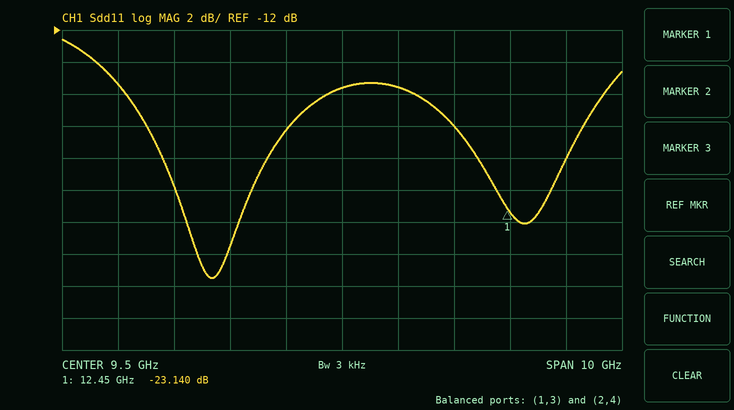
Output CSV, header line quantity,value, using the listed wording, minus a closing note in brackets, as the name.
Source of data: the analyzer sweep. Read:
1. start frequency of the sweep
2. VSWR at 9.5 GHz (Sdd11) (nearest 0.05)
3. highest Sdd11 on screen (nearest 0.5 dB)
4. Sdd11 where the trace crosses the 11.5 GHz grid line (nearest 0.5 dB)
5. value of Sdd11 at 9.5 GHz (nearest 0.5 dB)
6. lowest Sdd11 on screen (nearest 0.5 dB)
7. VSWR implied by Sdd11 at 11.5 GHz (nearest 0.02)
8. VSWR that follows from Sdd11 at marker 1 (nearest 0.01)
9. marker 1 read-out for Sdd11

quantity,value
start frequency of the sweep,4.5 GHz
VSWR at 9.5 GHz (Sdd11),1.40
highest Sdd11 on screen,-12.5 dB
Sdd11 where the trace crosses the 11.5 GHz grid line,-18.0 dB
value of Sdd11 at 9.5 GHz,-15.5 dB
lowest Sdd11 on screen,-27.5 dB
VSWR implied by Sdd11 at 11.5 GHz,1.28
VSWR that follows from Sdd11 at marker 1,1.15
marker 1 read-out for Sdd11,-23.140 dB
